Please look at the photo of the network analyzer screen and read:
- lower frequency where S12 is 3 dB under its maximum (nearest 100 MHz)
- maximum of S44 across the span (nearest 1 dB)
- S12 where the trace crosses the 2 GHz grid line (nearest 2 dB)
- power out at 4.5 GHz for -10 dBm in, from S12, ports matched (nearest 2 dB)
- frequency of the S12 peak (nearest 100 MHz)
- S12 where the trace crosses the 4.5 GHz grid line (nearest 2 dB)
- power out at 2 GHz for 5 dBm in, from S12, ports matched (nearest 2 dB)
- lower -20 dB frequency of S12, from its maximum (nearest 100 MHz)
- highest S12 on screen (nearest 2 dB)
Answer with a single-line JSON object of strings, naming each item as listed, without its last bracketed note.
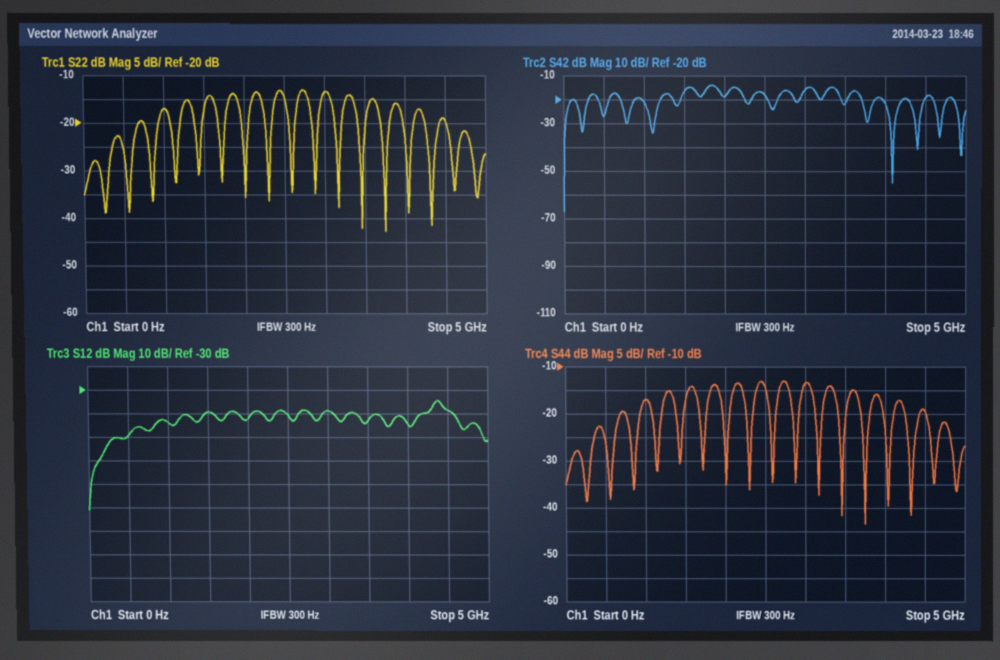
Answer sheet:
{"lower frequency where S12 is 3 dB under its maximum": "4.3 GHz", "maximum of S44 across the span": "-13 dB", "S12 where the trace crosses the 2 GHz grid line": "-42 dB", "power out at 4.5 GHz for -10 dBm in, from S12, ports matched": "-48 dBm", "frequency of the S12 peak": "4.4 GHz", "S12 where the trace crosses the 4.5 GHz grid line": "-38 dB", "power out at 2 GHz for 5 dBm in, from S12, ports matched": "-38 dBm", "lower -20 dB frequency of S12, from its maximum": "200 MHz", "highest S12 on screen": "-34 dB"}
